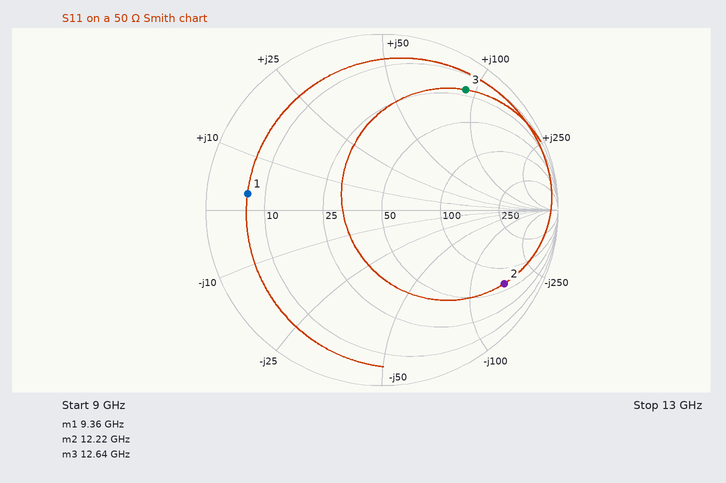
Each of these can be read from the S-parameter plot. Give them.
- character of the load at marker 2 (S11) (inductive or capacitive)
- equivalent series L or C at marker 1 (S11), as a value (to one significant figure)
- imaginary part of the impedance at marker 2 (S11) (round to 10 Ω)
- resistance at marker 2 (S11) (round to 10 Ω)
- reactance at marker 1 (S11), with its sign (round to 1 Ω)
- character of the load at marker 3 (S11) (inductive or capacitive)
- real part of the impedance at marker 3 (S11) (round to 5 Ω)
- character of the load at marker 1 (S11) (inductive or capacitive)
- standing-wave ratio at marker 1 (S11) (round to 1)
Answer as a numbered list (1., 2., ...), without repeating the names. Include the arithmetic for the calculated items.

1. capacitive
2. L = 3 Ω/(2π × 9.36 GHz) ≈ 51.0 pH, so 50 pH to one significant figure
3. -160 Ω
4. 60 Ω
5. +3 Ω
6. inductive
7. 20 Ω
8. inductive
9. 8
